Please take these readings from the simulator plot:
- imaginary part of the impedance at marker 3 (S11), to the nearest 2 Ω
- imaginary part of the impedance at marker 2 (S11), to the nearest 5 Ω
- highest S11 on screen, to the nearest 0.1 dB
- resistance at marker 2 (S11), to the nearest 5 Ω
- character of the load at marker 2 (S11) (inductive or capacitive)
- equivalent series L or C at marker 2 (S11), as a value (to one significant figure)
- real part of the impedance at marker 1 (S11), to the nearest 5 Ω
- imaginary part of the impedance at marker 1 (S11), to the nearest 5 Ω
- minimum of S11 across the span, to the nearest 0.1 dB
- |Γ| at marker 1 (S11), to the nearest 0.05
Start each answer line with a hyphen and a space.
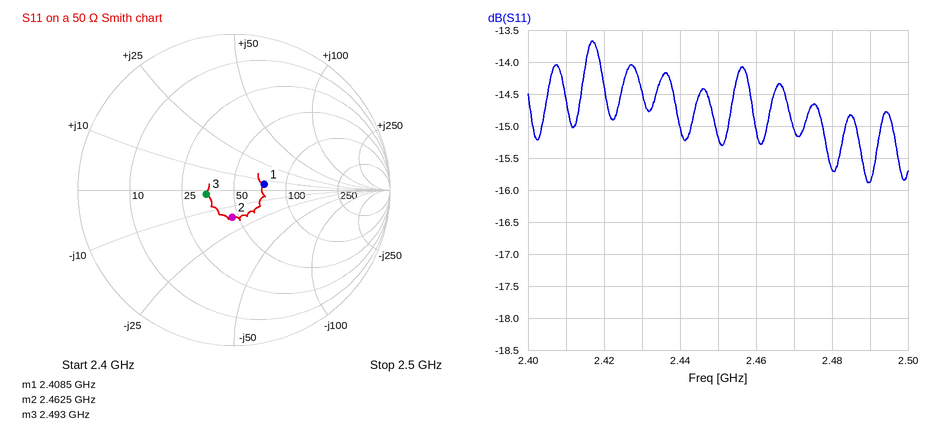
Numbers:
- -2 Ω
- -15 Ω
- -13.7 dB
- 45 Ω
- capacitive
- 4 pF
- 75 Ω
- +5 Ω
- -15.9 dB
- 0.20
